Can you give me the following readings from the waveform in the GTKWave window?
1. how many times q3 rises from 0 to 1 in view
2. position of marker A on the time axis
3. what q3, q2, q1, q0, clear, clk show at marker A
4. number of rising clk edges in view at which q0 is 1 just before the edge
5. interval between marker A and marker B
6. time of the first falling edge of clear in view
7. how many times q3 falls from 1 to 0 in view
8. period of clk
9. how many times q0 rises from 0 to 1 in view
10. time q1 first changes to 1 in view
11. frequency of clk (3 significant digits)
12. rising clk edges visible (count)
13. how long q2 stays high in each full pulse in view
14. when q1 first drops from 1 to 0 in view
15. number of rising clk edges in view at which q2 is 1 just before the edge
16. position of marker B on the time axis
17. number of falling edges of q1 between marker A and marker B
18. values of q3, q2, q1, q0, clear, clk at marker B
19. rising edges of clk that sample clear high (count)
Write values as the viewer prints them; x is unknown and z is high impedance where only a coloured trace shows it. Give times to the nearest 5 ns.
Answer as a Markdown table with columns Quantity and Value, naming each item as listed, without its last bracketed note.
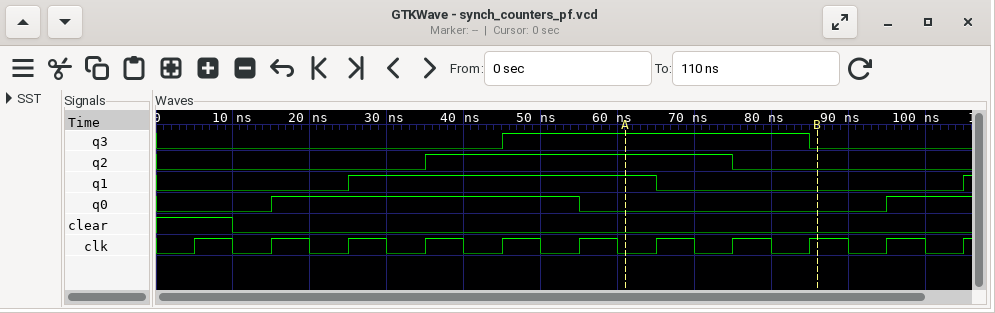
| Quantity | Value |
|---|---|
| how many times q3 rises from 0 to 1 in view | 1 |
| position of marker A on the time axis | 60 ns |
| what q3, q2, q1, q0, clear, clk show at marker A | q3=1, q2=1, q1=1, q0=0, clear=0, clk=0 |
| number of rising clk edges in view at which q0 is 1 just before the edge | 5 |
| interval between marker A and marker B | 25 ns |
| time of the first falling edge of clear in view | 10 ns |
| how many times q3 falls from 1 to 0 in view | 1 |
| period of clk | 10 ns |
| how many times q0 rises from 0 to 1 in view | 2 |
| time q1 first changes to 1 in view | 25 ns |
| frequency of clk | 100 MHz |
| rising clk edges visible | 11 |
| how long q2 stays high in each full pulse in view | 40 ns |
| when q1 first drops from 1 to 0 in view | 65 ns |
| number of rising clk edges in view at which q2 is 1 just before the edge | 4 |
| position of marker B on the time axis | 85 ns |
| number of falling edges of q1 between marker A and marker B | 1 |
| values of q3, q2, q1, q0, clear, clk at marker B | q3=0, q2=0, q1=0, q0=0, clear=0, clk=1 |
| rising edges of clk that sample clear high | 1 |
